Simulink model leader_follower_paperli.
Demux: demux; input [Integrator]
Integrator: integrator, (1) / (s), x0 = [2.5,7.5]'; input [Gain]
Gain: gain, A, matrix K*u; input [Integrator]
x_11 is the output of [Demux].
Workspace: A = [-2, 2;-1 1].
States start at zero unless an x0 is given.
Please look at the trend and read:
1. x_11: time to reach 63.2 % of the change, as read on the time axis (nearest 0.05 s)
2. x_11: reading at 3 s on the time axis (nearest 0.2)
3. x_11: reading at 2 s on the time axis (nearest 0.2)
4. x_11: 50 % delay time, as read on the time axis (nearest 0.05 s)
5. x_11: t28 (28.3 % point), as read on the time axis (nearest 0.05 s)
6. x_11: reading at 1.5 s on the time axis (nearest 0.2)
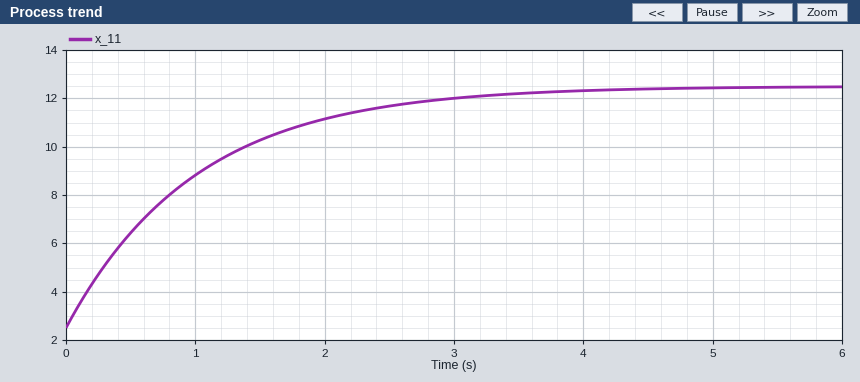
1.00 s
12.0
11.2
0.70 s
0.35 s
10.2
